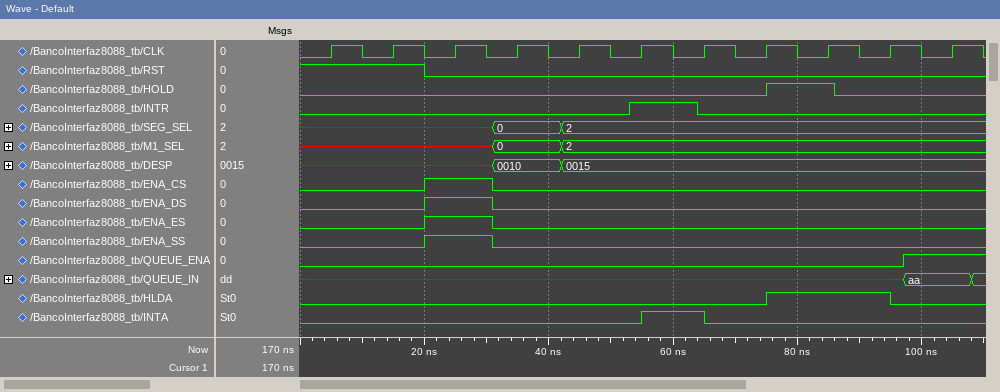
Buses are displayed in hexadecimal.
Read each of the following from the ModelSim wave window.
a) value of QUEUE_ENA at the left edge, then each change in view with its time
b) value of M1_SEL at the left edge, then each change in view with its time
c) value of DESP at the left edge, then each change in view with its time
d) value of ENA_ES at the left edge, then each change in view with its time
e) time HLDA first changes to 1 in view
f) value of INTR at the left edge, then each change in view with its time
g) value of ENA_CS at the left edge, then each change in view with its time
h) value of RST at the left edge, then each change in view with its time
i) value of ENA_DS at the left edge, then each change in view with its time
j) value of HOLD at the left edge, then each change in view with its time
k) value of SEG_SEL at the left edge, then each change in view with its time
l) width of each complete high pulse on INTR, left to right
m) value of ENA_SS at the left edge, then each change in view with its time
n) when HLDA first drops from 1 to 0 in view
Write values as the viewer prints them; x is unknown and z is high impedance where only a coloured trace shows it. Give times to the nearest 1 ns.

0, 1 at 97 ns
x, 0 at 31 ns, 2 at 42 ns
x, 0010 at 31 ns, 0015 at 42 ns
0, 1 at 20 ns, 0 at 31 ns
75 ns
0, 1 at 53 ns, 0 at 64 ns
0, 1 at 20 ns, 0 at 31 ns
1, 0 at 20 ns
0, 1 at 20 ns, 0 at 31 ns
0, 1 at 75 ns, 0 at 86 ns
x, 0 at 31 ns, 2 at 42 ns
11 ns
0, 1 at 20 ns, 0 at 31 ns
95 ns
